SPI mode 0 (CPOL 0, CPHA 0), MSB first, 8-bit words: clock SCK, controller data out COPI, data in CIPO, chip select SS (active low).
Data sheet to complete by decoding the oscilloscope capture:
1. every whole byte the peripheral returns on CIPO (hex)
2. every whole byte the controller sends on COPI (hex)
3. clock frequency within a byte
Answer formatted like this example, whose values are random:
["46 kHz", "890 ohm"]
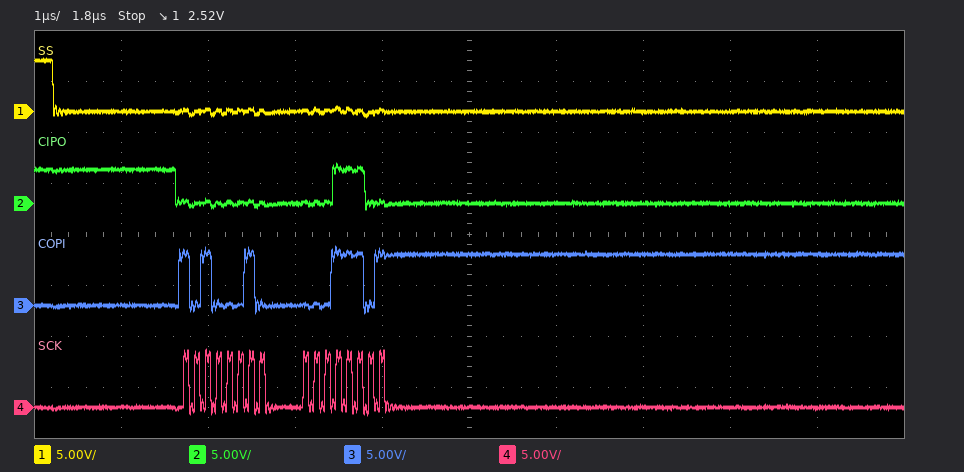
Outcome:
["0x00 0x1C", "0xA2 0x1D", "8 MHz"]
